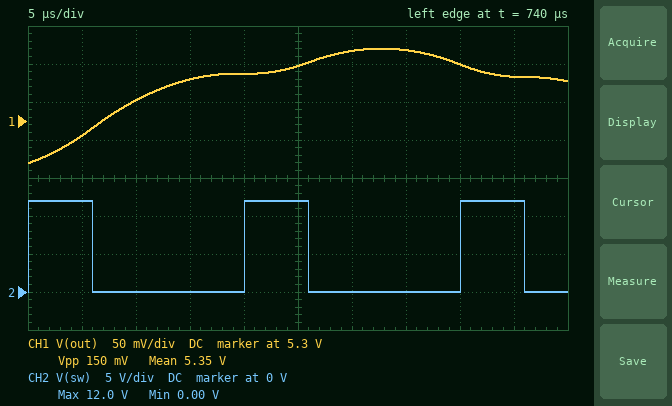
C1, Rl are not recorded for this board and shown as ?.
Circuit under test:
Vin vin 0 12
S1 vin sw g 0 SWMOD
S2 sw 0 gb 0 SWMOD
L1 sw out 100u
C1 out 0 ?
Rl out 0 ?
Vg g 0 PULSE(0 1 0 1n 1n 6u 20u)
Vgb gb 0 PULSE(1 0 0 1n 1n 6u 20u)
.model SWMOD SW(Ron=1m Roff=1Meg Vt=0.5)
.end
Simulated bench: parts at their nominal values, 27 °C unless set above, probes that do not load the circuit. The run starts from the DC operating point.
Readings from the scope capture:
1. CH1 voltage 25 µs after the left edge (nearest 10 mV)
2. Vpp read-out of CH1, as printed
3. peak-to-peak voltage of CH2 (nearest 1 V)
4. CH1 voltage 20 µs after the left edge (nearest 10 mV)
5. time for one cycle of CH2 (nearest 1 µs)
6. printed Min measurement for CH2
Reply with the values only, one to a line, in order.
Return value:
5.37 V
150 mV
12 V
5.36 V
20 µs
0.00 V
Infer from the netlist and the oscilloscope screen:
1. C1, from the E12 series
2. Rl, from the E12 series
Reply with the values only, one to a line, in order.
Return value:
68 µF
8.2 Ω
